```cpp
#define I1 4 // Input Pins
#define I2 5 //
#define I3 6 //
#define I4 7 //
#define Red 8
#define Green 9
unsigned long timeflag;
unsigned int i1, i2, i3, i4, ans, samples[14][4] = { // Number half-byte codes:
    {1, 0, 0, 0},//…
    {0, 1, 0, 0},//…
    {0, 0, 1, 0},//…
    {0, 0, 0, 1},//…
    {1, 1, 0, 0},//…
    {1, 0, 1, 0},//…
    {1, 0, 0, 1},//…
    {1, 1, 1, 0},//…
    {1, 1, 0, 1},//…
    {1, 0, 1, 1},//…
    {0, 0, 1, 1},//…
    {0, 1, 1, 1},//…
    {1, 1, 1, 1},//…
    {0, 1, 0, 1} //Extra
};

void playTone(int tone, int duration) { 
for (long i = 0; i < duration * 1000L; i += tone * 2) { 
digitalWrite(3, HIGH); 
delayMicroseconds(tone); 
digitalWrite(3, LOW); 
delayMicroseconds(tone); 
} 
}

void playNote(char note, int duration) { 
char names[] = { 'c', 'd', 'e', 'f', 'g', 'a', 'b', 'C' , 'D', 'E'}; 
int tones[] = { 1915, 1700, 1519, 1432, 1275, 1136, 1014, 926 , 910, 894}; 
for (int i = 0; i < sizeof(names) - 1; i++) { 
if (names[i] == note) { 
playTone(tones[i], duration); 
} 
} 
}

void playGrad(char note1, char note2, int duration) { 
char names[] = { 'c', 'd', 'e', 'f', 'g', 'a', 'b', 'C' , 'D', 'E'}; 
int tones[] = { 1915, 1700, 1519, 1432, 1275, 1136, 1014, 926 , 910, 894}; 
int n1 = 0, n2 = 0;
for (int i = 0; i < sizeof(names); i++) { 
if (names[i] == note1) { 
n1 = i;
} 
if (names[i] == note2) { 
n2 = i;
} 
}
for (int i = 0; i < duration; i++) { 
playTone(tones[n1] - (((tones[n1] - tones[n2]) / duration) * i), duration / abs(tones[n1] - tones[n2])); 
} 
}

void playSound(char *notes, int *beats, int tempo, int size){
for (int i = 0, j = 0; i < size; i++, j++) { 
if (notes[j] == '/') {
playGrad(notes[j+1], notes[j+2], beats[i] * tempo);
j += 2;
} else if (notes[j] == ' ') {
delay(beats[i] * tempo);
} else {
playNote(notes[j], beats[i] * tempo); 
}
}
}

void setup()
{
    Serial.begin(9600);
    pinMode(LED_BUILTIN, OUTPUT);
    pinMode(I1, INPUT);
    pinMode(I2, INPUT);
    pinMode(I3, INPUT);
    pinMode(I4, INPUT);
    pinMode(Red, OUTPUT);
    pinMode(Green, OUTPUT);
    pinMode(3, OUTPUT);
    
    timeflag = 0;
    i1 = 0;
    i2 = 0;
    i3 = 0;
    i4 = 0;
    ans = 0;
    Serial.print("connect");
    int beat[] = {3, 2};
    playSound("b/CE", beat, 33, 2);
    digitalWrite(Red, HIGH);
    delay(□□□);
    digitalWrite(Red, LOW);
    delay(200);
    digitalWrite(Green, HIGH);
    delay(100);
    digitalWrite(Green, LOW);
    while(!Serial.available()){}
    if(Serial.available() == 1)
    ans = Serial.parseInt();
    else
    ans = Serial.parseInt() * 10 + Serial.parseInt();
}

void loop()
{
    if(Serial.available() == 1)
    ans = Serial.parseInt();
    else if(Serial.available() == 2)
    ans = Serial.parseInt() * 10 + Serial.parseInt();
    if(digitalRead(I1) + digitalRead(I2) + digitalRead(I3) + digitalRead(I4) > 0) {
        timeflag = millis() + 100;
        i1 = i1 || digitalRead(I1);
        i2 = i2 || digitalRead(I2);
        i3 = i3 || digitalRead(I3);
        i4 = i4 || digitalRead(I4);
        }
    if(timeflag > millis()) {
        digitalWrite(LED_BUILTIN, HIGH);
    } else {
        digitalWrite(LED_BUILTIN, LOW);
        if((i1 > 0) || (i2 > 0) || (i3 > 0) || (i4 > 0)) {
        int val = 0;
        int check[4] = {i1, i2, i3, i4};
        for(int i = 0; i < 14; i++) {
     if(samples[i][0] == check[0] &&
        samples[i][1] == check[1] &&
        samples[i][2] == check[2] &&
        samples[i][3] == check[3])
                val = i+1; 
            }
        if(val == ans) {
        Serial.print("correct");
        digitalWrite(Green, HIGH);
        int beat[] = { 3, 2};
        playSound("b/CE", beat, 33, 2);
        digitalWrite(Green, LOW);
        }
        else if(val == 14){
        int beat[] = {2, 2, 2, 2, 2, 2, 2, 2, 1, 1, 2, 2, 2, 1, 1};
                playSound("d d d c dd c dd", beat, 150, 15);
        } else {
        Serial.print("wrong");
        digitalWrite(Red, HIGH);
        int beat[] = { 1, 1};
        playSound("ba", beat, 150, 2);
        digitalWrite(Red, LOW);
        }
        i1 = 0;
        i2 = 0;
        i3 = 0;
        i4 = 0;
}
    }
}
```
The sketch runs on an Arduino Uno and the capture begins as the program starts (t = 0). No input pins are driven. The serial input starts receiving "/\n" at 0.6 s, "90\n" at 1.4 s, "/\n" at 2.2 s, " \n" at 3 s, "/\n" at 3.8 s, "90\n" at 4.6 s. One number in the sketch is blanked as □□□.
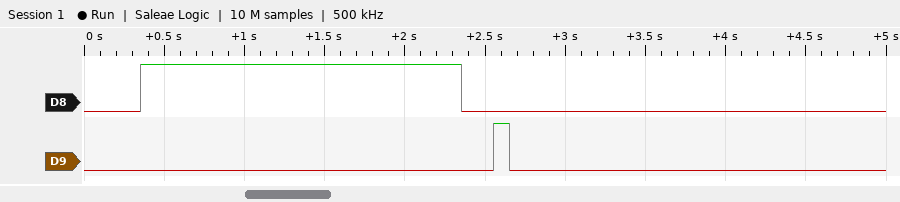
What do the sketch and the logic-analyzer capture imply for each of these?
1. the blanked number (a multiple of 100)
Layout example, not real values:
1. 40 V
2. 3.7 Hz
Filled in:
1. 2000
